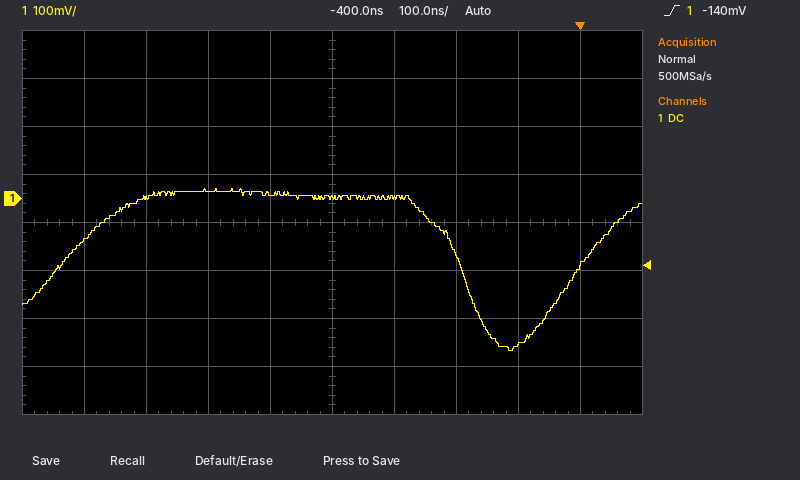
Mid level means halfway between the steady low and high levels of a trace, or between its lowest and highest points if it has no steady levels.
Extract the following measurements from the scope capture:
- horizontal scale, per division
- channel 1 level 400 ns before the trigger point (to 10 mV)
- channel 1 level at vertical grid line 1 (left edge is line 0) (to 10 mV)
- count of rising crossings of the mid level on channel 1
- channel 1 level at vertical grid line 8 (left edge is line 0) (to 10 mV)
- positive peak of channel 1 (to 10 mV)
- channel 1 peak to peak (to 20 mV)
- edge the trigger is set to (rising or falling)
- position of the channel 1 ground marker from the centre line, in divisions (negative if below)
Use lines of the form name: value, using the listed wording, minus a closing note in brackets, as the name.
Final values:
horizontal scale, per division: 100 ns
channel 1 level 400 ns before the trigger point: 0 mV
channel 1 level at vertical grid line 1 (left edge is line 0): -90 mV
count of rising crossings of the mid level on channel 1: 2
channel 1 level at vertical grid line 8 (left edge is line 0): -300 mV
positive peak of channel 1: 20 mV
channel 1 peak to peak: 340 mV
edge the trigger is set to: rising
position of the channel 1 ground marker from the centre line, in divisions: +0.5 div
